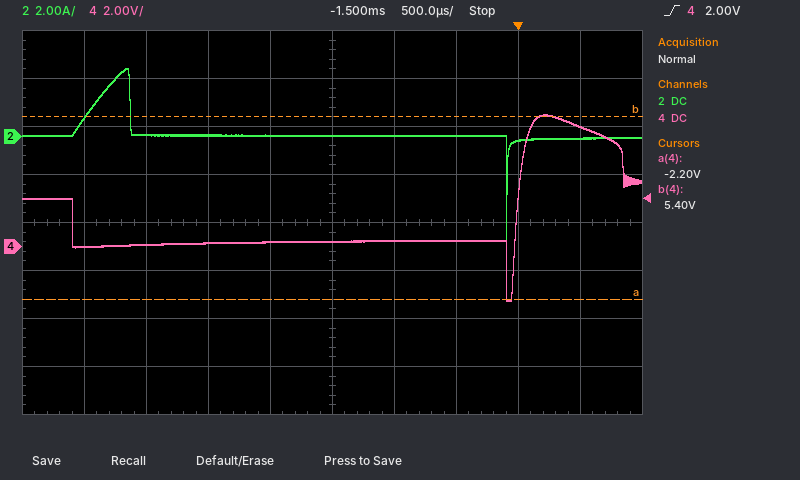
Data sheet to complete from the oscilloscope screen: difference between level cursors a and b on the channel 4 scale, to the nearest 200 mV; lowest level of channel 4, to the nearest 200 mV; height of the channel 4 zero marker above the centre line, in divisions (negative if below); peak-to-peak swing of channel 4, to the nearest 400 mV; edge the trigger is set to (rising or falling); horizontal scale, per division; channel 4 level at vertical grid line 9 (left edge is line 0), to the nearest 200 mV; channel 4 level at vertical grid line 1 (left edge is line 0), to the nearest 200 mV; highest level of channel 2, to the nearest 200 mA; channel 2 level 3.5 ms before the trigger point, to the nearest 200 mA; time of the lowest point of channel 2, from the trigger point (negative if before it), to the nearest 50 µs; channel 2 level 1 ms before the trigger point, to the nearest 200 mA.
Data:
7.6 V
-2.2 V
-0.5 div
7.6 V
rising
500 µs
5.0 V
0.0 V
2.8 A
800 mA
-100 µs
0.0 A
